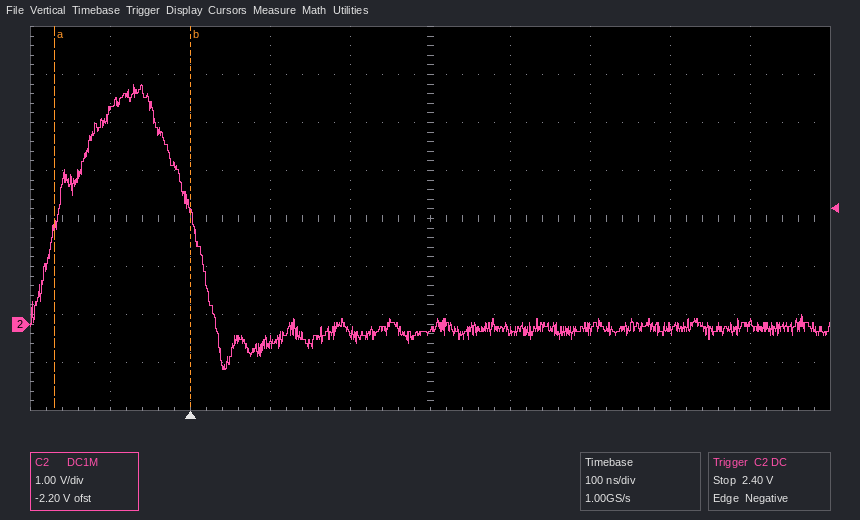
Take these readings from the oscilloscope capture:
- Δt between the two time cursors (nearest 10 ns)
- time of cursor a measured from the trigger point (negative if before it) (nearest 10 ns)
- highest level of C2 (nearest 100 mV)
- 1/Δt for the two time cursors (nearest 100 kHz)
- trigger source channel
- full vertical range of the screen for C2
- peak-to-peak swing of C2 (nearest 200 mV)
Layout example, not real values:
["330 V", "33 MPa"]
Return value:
["170 ns", "-170 ns", "5.0 V", "5.9 MHz", "C2", "8 V", "6.0 V"]
